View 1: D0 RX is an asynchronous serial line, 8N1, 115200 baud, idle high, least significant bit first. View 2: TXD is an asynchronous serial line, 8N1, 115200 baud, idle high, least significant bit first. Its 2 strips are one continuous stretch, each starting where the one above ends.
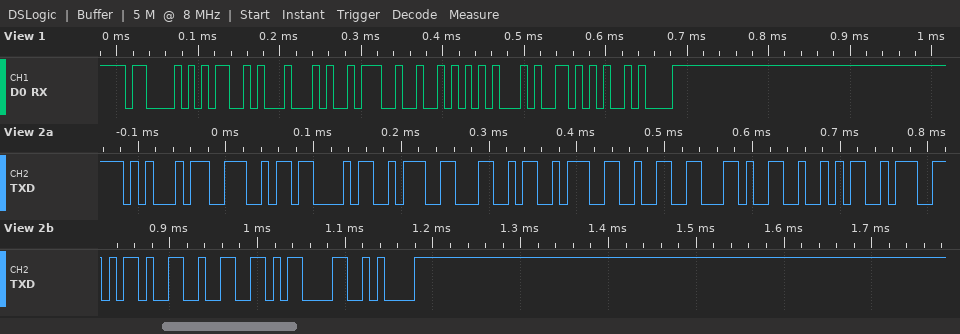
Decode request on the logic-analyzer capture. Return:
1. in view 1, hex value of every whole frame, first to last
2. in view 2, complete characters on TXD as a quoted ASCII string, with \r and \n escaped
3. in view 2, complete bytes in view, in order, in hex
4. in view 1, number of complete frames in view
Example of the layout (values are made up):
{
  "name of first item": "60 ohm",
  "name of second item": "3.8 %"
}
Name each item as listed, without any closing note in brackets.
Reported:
{
  "in view 1, hex value of every whole frame, first to last": "0x43 0x4D 0x44 0x3A 0x52 0x45 0x56 0x0A",
  "in view 2, complete characters on TXD as a quoted ASCII string, with \\r and \\n escaped": "\"ENC:L:2,R:-2\\r\\n\"",
  "in view 2, complete bytes in view, in order, in hex": "45 4E 43 3A 4C 3A 32 2C 52 3A 2D 32 0D 0A",
  "in view 1, number of complete frames in view": "8"
}
